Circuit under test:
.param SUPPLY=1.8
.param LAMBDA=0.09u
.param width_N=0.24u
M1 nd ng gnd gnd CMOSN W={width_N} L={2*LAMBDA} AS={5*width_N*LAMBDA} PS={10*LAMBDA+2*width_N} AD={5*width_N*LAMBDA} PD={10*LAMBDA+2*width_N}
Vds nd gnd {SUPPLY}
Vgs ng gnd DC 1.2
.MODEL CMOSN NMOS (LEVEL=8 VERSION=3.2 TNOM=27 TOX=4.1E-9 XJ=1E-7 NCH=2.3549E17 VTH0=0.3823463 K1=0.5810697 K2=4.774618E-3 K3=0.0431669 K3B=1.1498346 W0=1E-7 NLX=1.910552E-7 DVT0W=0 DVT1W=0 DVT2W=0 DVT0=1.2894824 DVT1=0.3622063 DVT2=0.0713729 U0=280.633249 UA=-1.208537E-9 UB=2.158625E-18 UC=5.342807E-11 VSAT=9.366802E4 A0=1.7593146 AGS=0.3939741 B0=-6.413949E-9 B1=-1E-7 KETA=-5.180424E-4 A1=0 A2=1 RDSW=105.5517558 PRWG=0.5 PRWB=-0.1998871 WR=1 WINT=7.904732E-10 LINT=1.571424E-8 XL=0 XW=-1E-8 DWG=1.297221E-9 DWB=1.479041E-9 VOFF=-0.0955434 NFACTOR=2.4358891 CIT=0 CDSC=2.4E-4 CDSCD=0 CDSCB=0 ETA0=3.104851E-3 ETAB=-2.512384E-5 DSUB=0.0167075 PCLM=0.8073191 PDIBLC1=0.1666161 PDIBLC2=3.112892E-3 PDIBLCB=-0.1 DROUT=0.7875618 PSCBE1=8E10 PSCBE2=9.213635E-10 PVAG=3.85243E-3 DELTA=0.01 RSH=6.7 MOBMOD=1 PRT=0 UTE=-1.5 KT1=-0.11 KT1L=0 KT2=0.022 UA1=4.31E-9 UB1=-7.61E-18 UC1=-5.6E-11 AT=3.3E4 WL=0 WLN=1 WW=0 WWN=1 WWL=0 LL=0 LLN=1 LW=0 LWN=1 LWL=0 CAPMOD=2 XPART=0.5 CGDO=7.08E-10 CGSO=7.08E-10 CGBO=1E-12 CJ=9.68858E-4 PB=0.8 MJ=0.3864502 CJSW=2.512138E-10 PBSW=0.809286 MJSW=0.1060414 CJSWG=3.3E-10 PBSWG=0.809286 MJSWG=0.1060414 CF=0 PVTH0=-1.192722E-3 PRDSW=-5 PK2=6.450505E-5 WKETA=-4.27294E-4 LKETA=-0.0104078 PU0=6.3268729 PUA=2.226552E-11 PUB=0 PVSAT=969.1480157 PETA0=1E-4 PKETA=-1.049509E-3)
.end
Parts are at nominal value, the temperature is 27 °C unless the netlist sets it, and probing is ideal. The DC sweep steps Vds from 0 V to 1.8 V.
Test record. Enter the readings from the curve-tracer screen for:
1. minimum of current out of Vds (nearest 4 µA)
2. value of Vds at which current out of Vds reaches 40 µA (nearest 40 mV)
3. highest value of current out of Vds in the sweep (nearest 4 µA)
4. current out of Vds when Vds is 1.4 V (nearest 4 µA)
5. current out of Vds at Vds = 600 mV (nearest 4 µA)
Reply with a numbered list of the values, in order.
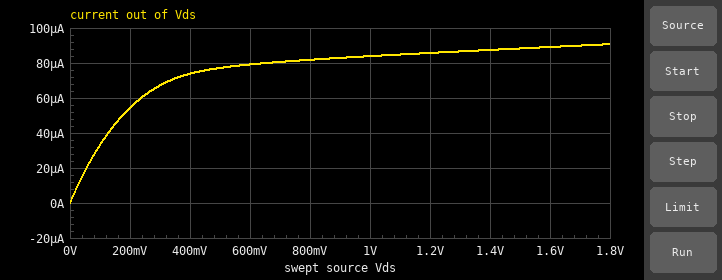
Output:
1. 0 A
2. 120 mV
3. 92 µA
4. 88 µA
5. 80 µA
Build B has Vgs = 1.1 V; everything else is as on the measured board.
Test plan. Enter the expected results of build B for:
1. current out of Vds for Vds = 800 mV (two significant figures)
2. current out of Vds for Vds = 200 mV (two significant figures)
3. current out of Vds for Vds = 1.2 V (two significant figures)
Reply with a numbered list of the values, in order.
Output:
1. 66 µA
2. 46 µA
3. 70 µA
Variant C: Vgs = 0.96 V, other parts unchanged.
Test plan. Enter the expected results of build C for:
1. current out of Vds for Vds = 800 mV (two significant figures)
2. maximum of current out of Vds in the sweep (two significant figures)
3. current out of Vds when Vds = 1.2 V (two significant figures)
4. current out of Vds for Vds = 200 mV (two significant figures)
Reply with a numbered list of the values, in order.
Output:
1. 46 µA
2. 53 µA
3. 49 µA
4. 34 µA
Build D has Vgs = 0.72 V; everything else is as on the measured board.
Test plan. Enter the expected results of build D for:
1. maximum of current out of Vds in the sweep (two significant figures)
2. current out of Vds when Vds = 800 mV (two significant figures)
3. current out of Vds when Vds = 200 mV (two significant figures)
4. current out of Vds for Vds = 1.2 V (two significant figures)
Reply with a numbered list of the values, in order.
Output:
1. 20 µA
2. 16 µA
3. 12 µA
4. 18 µA
